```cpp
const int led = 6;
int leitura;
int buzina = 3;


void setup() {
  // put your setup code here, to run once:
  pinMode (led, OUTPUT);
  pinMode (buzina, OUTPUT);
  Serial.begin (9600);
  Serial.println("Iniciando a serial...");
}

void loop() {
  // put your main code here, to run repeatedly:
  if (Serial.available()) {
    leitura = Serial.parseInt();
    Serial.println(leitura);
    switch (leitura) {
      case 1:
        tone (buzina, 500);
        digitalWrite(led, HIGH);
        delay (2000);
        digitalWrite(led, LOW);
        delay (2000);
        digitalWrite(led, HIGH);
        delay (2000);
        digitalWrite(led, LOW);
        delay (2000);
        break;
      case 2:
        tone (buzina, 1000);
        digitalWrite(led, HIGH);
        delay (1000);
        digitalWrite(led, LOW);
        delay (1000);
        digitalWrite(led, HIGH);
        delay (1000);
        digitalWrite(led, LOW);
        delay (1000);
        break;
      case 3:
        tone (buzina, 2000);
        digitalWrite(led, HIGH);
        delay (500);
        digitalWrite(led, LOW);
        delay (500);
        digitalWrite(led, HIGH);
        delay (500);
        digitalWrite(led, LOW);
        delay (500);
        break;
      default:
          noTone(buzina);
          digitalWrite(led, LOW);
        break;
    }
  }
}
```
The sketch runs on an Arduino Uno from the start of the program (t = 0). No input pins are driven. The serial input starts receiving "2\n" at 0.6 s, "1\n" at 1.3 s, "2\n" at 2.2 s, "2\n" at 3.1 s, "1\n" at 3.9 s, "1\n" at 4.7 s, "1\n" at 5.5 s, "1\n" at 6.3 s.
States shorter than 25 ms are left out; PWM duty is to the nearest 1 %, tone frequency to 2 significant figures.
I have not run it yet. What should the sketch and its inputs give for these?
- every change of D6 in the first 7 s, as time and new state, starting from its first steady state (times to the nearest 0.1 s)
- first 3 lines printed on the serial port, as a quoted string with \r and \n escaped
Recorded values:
0 s low; 0.6 s high; 1.6 s low; 2.6 s high; 3.6 s low; 4.6 s high; 6.6 s low
"Iniciando a serial...\r\n2\r\n1\r\n"
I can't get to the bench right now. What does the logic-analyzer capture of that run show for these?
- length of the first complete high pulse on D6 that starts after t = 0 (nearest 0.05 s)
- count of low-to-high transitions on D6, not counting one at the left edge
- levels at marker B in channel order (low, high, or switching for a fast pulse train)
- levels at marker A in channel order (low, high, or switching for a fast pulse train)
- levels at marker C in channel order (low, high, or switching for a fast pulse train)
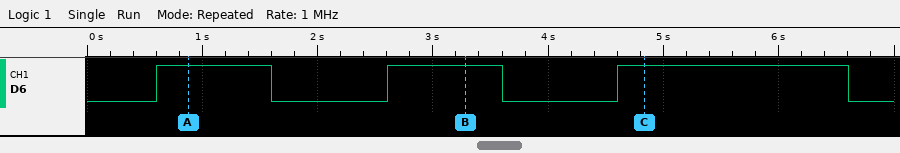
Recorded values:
1.00 s
3
D6 high
D6 high
D6 high
